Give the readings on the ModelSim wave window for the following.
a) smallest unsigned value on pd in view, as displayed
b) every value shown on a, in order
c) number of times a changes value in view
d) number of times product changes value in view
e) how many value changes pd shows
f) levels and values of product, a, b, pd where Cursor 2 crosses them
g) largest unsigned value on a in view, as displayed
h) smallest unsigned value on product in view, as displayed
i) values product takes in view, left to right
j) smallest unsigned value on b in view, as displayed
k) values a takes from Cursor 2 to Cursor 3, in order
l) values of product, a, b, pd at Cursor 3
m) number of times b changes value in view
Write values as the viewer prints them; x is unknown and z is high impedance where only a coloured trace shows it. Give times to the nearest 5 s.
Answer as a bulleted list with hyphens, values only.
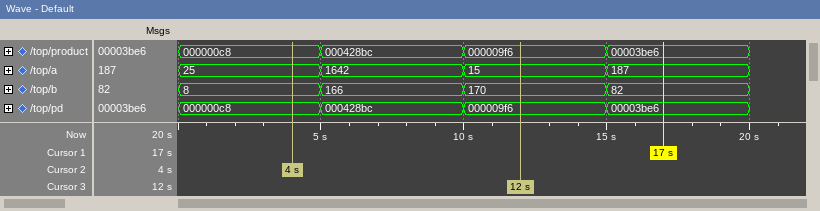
- 000000c8
- 25, 1642, 15, 187
- 3
- 3
- 3
- product=000000c8, a=25, b=8, pd=000000c8
- 1642
- 000000c8
- 000000c8, 000428bc, 000009f6, 00003be6
- 8
- 25, 1642, 15
- product=000009f6, a=15, b=170, pd=000009f6
- 3
